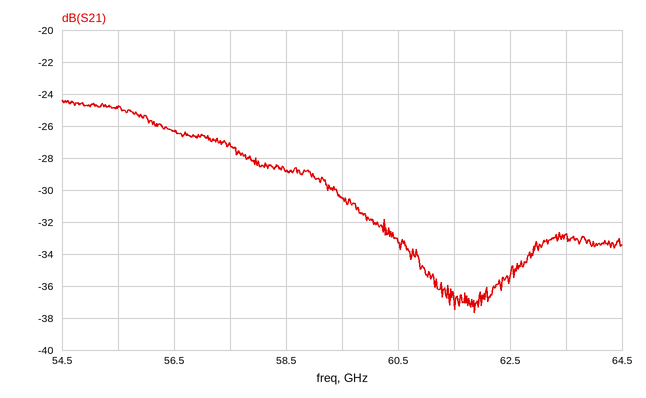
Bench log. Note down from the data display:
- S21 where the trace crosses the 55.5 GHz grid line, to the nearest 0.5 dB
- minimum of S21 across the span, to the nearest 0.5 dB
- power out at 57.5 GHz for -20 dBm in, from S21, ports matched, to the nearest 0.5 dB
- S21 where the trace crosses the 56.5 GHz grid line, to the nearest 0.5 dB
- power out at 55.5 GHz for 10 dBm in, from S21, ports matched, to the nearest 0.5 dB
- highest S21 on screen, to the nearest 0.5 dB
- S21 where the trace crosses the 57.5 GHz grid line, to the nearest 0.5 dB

-25.0 dB
-37.5 dB
-47.0 dBm
-26.5 dB
-15.0 dBm
-24.5 dB
-27.0 dB
